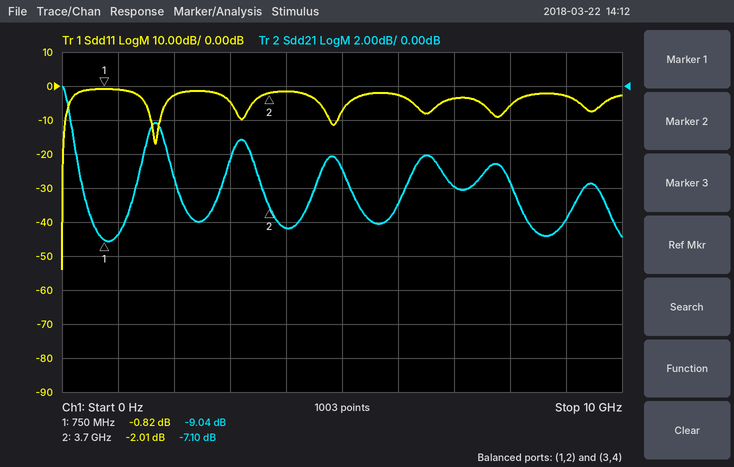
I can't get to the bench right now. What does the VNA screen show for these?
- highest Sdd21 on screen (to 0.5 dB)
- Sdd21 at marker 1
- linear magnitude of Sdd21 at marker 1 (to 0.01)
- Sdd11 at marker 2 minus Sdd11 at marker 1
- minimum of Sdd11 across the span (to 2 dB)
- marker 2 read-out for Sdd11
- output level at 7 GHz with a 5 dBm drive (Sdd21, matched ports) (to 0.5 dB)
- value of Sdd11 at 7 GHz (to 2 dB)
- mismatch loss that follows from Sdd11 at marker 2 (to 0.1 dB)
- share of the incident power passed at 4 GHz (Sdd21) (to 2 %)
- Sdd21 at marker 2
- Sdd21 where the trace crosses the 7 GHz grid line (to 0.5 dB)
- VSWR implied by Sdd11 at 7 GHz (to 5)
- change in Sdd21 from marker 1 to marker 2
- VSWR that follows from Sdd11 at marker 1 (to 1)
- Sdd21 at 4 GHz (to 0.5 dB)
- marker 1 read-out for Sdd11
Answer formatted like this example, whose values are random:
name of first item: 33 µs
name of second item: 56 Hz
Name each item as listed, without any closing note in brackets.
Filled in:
highest Sdd21 on screen: 0.0 dB
Sdd21 at marker 1: -9.04 dB
linear magnitude of Sdd21 at marker 1: 0.35
Sdd11 at marker 2 minus Sdd11 at marker 1: -1.19 dB
minimum of Sdd11 across the span: -54 dB
marker 2 read-out for Sdd11: -2.01 dB
output level at 7 GHz with a 5 dBm drive (Sdd21, matched ports): -1.0 dBm
value of Sdd11 at 7 GHz: -4 dB
mismatch loss that follows from Sdd11 at marker 2: 4.3 dB
share of the incident power passed at 4 GHz (Sdd21): 14 %
Sdd21 at marker 2: -7.10 dB
Sdd21 where the trace crosses the 7 GHz grid line: -6.0 dB
VSWR implied by Sdd11 at 7 GHz: 5
change in Sdd21 from marker 1 to marker 2: 1.94 dB
VSWR that follows from Sdd11 at marker 1: 21
Sdd21 at 4 GHz: -8.5 dB
marker 1 read-out for Sdd11: -0.82 dB
